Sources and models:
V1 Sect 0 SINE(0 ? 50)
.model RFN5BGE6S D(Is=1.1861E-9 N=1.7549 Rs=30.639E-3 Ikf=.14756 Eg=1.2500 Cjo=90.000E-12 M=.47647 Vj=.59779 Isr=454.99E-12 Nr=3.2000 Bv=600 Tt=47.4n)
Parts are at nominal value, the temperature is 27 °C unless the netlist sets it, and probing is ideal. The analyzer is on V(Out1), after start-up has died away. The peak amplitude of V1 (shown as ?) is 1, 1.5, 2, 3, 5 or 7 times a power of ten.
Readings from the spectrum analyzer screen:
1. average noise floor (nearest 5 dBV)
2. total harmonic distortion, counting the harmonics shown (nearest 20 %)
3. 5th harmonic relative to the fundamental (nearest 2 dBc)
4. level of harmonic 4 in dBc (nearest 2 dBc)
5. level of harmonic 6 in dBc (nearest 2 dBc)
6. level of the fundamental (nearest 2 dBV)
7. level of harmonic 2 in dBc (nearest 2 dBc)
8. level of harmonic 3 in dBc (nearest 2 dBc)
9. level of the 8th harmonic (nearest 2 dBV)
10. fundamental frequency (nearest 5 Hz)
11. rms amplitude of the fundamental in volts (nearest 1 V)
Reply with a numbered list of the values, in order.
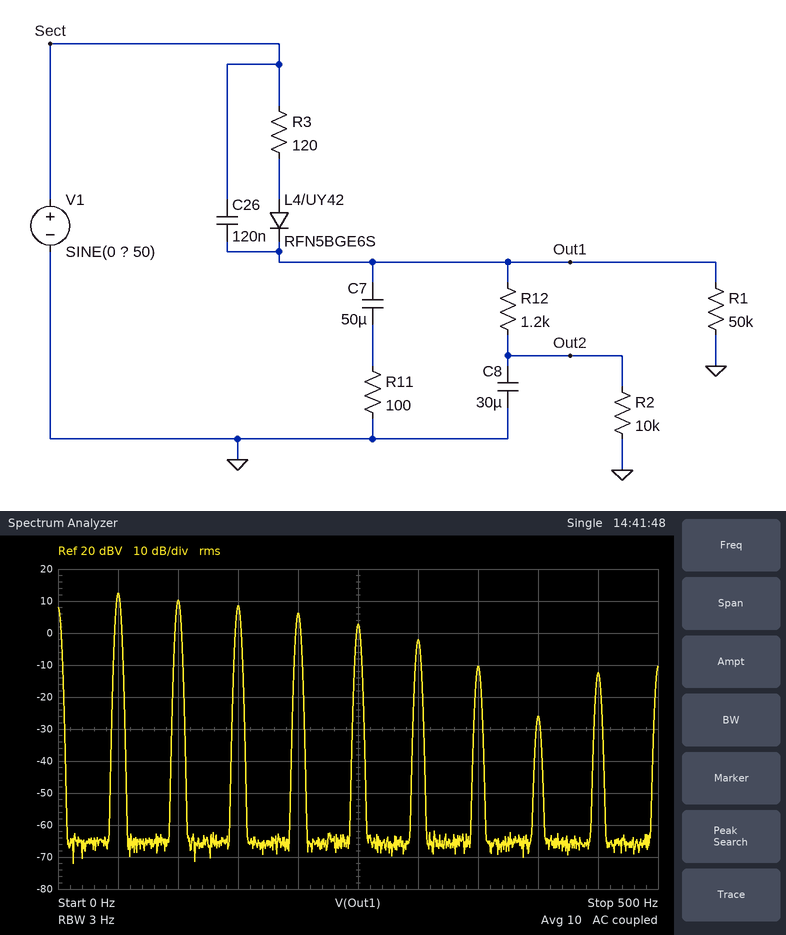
1. -65 dBV
2. 120 %
3. -10 dBc
4. -6 dBc
5. -14 dBc
6. 12 dBV
7. -2 dBc
8. -4 dBc
9. -26 dBV
10. 50 Hz
11. 4 V
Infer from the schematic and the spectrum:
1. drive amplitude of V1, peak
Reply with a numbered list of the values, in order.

1. 300 V
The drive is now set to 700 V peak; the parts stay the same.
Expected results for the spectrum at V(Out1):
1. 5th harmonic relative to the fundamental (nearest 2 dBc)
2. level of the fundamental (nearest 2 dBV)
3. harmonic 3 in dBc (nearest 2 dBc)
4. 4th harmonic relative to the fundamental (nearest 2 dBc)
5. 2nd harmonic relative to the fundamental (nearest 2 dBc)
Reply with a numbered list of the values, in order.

1. -22 dBc
2. 42 dBV
3. -12 dBc
4. -42 dBc
5. -38 dBc
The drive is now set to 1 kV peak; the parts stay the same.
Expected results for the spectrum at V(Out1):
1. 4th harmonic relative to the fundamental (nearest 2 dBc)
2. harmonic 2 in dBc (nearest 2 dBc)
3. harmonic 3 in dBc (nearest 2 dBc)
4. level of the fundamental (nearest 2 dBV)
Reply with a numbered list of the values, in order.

1. -48 dBc
2. -46 dBc
3. -16 dBc
4. 46 dBV
